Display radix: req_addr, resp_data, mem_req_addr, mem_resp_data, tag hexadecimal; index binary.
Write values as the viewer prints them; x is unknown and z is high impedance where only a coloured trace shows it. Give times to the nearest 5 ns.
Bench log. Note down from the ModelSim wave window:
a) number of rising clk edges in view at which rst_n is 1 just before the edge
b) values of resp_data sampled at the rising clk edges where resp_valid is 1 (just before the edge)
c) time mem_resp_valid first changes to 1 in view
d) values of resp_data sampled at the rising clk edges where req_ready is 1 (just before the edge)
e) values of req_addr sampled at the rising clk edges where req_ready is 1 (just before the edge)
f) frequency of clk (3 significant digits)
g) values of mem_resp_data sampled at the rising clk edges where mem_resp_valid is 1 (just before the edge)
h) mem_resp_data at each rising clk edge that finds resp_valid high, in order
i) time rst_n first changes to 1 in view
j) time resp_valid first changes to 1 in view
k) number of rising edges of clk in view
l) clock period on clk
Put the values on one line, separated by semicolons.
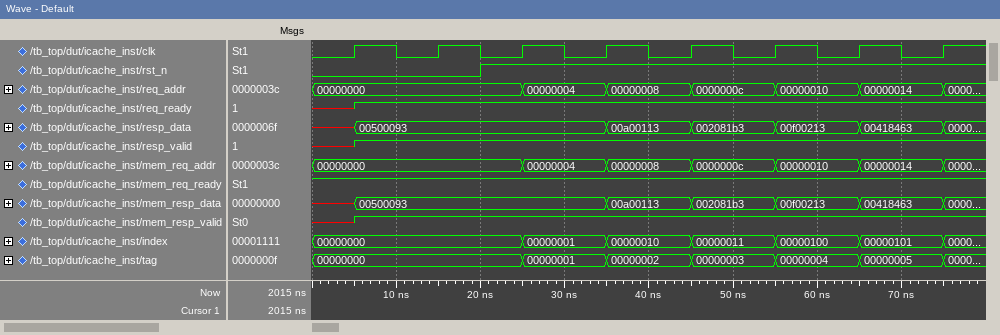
6; 00500093, 00500093, 00500093, 00a00113, 002081b3, 00f00213, 00418463; 5 ns; 00500093, 00500093, 00500093, 00a00113, 002081b3, 00f00213, 00418463; 00000000, 00000000, 00000004, 00000008, 0000000c, 00000010, 00000014; 100 MHz; 00500093, 00500093, 00500093, 00a00113, 002081b3, 00f00213, 00418463; 00500093, 00500093, 00500093, 00a00113, 002081b3, 00f00213, 00418463; 20 ns; 5 ns; 8; 10 ns
